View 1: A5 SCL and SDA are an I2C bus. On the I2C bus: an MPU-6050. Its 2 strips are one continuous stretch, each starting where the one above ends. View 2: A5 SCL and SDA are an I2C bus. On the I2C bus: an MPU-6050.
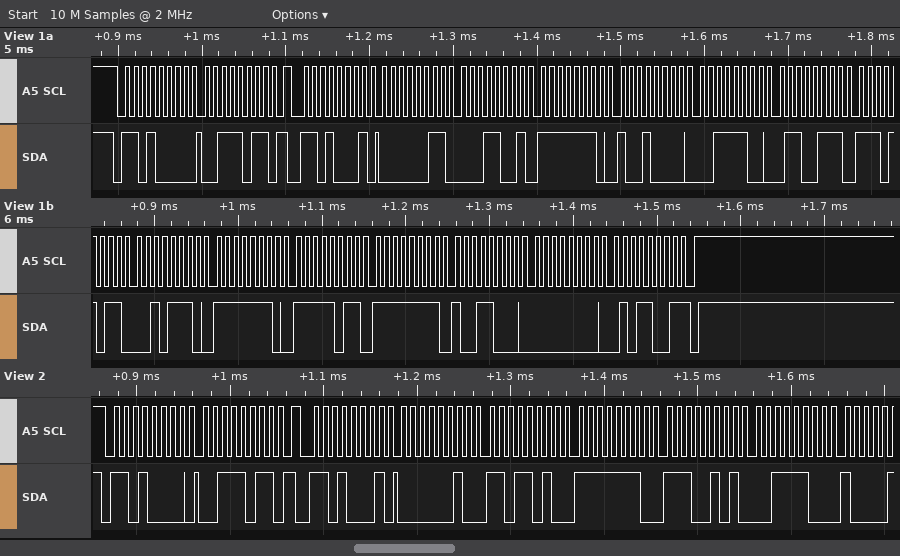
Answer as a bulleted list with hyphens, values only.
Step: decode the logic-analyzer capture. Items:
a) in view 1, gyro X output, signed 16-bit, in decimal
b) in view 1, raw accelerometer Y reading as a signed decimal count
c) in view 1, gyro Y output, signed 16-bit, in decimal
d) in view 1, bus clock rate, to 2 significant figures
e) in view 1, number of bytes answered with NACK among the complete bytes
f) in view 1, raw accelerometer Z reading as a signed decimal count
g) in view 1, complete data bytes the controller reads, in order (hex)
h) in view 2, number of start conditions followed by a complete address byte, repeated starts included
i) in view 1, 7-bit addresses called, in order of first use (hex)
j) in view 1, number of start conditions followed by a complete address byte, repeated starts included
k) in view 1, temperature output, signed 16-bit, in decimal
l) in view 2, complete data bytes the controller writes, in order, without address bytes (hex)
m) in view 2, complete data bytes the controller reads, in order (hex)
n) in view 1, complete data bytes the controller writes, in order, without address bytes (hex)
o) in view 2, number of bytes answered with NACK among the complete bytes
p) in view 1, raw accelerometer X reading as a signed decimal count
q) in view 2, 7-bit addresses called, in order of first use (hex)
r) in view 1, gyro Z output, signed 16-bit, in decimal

- -261
- -368
- -104
- 100 kHz
- 1
- 15463
- 03 19 FE 90 3C 67 EB 2E FE FB FF 98 00 59
- 2
- 0x68
- 2
- -5330
- 3B
- 02 DA FE E5 3C
- 3B
- 0
- 793
- 0x68
- 89
